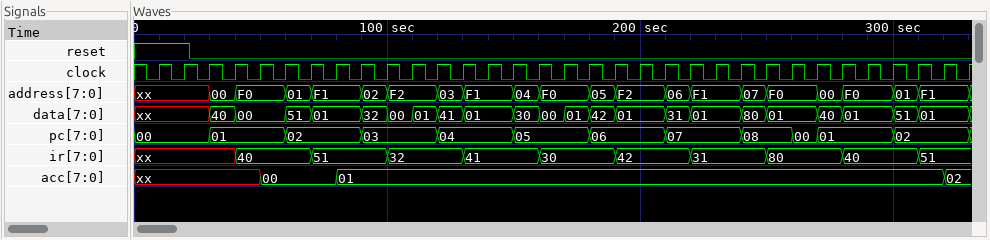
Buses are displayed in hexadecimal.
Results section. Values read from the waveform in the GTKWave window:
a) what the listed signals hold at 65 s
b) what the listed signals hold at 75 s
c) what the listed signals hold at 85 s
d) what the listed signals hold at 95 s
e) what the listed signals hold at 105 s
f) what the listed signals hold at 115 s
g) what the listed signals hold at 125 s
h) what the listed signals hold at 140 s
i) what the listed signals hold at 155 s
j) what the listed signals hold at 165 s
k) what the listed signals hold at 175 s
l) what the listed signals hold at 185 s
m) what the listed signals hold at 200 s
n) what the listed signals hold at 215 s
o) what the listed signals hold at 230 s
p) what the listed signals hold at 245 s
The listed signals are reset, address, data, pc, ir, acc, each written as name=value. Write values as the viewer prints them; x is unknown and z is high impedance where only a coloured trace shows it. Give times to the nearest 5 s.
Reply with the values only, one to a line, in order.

reset=0, address=01, data=51, pc=02, ir=40, acc=00
reset=0, address=F1, data=01, pc=02, ir=51, acc=00
reset=0, address=F1, data=01, pc=02, ir=51, acc=01
reset=0, address=02, data=32, pc=03, ir=51, acc=01
reset=0, address=F2, data=00, pc=03, ir=32, acc=01
reset=0, address=F2, data=01, pc=03, ir=32, acc=01
reset=0, address=03, data=41, pc=04, ir=32, acc=01
reset=0, address=F1, data=01, pc=04, ir=41, acc=01
reset=0, address=04, data=30, pc=05, ir=41, acc=01
reset=0, address=F0, data=00, pc=05, ir=30, acc=01
reset=0, address=F0, data=01, pc=05, ir=30, acc=01
reset=0, address=05, data=42, pc=06, ir=30, acc=01
reset=0, address=F2, data=01, pc=06, ir=42, acc=01
reset=0, address=06, data=31, pc=07, ir=42, acc=01
reset=0, address=F1, data=01, pc=07, ir=31, acc=01
reset=0, address=07, data=80, pc=08, ir=31, acc=01
